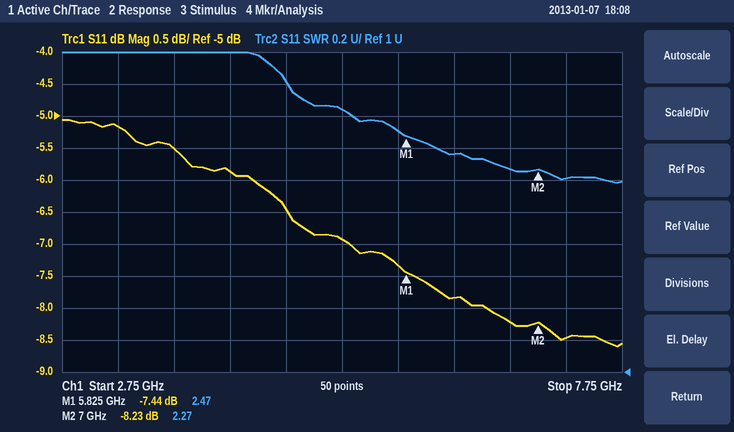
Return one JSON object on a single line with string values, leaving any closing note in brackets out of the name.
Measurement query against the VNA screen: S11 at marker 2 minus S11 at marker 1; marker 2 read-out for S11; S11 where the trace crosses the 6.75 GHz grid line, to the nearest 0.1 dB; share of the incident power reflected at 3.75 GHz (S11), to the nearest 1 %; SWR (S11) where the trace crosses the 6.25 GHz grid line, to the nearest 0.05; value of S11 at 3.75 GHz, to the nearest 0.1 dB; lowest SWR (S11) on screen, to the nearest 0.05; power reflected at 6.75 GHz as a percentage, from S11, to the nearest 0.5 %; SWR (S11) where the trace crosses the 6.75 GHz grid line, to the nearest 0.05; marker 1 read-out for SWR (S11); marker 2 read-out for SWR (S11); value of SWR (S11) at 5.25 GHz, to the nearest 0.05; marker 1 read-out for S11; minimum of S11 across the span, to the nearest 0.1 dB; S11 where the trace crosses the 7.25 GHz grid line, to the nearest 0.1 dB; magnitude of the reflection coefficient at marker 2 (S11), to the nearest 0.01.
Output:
{"S11 at marker 2 minus S11 at marker 1": "-0.79 dB", "marker 2 read-out for S11": "-8.23 dB", "S11 where the trace crosses the 6.75 GHz grid line, to the nearest 0.1 dB": "-8.2 dB", "share of the incident power reflected at 3.75 GHz (S11), to the nearest 1 %": "28 %", "SWR (S11) where the trace crosses the 6.25 GHz grid line, to the nearest 0.05": "2.35", "value of S11 at 3.75 GHz, to the nearest 0.1 dB": "-5.5 dB", "lowest SWR (S11) on screen, to the nearest 0.05": "2.20", "power reflected at 6.75 GHz as a percentage, from S11, to the nearest 0.5 %": "15.0 %", "SWR (S11) where the trace crosses the 6.75 GHz grid line, to the nearest 0.05": "2.25", "marker 1 read-out for SWR": "2.47", "marker 2 read-out for SWR": "2.27", "value of SWR (S11) at 5.25 GHz, to the nearest 0.05": "2.65", "marker 1 read-out for S11": "-7.44 dB", "minimum of S11 across the span, to the nearest 0.1 dB": "-8.6 dB", "S11 where the trace crosses the 7.25 GHz grid line, to the nearest 0.1 dB": "-8.5 dB", "magnitude of the reflection coefficient at marker 2 (S11), to the nearest 0.01": "0.39"}
